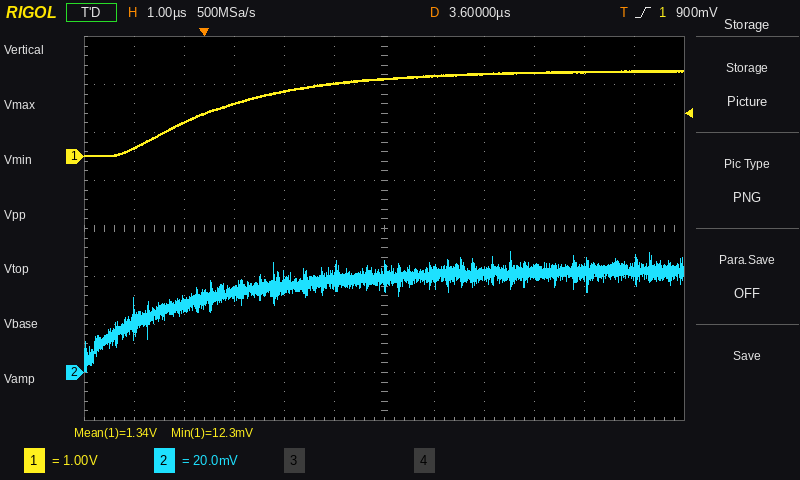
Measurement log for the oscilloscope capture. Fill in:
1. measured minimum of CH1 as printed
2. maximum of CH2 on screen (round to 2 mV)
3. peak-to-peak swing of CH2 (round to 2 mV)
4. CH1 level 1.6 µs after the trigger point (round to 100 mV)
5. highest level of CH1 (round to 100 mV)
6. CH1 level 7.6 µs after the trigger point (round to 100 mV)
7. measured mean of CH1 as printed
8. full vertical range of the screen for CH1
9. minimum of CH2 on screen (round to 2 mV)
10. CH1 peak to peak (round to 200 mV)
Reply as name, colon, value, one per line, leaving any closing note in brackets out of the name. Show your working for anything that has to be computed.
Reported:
measured minimum of CH1 as printed: 12.3 mV
maximum of CH2 on screen: 50 mV
peak-to-peak swing of CH2: 50 mV − (0 mV) = 50 mV
CH1 level 1.6 µs after the trigger point: 1.4 V
highest level of CH1: 1.8 V
CH1 level 7.6 µs after the trigger point: 1.8 V
measured mean of CH1 as printed: 1.34 V
full vertical range of the screen for CH1: 8 V
minimum of CH2 on screen: 0 mV
CH1 peak to peak: 1.8 V
